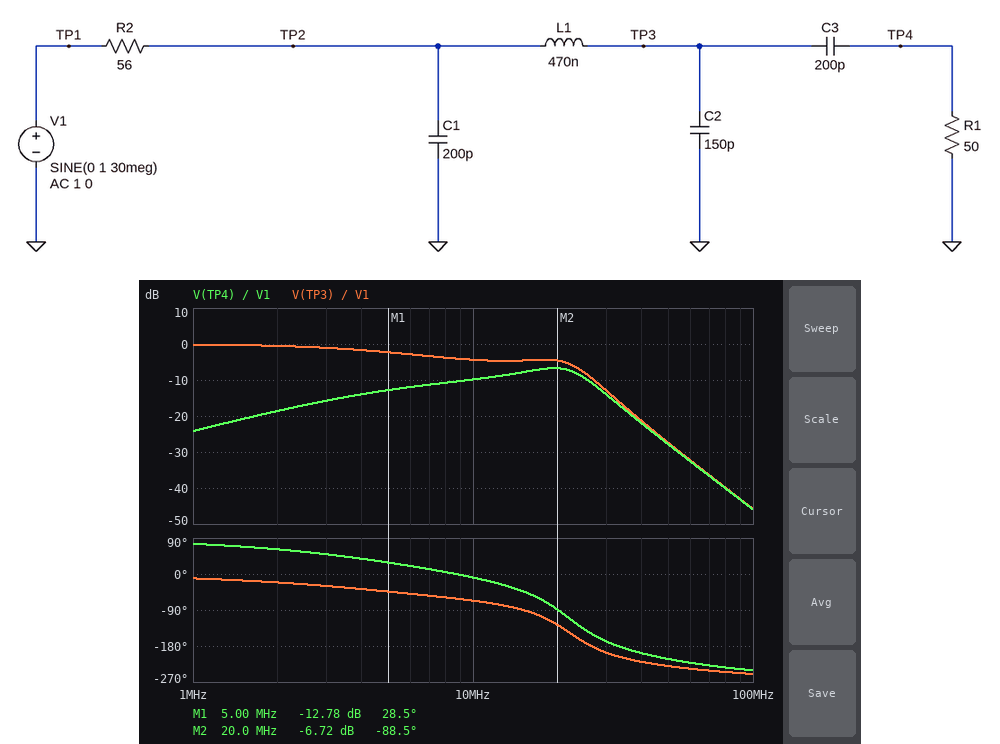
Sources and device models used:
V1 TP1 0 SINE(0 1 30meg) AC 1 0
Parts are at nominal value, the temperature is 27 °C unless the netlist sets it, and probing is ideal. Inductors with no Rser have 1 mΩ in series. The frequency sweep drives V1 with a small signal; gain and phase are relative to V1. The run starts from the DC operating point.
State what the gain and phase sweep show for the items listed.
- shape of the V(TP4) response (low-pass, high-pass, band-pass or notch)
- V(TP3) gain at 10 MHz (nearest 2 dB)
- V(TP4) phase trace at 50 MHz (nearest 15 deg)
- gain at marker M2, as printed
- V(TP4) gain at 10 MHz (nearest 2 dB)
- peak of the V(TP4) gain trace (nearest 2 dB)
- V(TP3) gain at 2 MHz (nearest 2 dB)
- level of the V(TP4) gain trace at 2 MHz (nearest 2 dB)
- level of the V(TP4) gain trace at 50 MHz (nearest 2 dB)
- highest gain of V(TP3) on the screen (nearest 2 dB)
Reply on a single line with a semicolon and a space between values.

band-pass; -4 dB; -210 deg; -6.72 dB; -10 dB; -6 dB; 0 dB; -18 dB; -28 dB; 0 dB
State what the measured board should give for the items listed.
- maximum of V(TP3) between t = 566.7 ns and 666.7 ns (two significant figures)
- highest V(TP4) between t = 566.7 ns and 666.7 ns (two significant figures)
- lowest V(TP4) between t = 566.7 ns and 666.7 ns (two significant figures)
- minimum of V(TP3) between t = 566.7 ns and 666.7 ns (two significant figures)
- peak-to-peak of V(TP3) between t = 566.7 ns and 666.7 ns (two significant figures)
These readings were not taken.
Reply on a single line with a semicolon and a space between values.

220 mV; 200 mV; -200 mV; -220 mV; 450 mV
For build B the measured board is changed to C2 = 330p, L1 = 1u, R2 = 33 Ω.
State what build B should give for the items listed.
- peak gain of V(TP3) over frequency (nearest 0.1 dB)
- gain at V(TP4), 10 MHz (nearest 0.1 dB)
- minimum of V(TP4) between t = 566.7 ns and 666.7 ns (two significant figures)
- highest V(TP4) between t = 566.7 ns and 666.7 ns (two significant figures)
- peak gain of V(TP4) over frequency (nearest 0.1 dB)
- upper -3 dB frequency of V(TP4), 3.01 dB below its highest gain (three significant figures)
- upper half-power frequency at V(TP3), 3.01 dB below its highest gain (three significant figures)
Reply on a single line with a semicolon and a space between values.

1.3 dB; -7.6 dB; -48 mV; 48 mV; -6.5 dB; 11.8 MHz; 9.72 MHz
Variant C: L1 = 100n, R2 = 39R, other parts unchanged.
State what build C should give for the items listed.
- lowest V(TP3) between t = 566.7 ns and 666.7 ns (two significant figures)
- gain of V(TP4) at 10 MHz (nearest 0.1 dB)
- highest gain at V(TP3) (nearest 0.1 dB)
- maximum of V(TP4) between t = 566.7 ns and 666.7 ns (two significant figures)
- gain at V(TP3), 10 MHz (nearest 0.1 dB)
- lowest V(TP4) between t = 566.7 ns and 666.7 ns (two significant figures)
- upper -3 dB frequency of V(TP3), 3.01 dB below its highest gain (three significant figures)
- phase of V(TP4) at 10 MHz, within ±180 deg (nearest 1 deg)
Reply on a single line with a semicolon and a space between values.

-450 mV; -9.6 dB; 0 dB; 400 mV; -4.1 dB; -400 mV; 7.45 MHz; 10 deg
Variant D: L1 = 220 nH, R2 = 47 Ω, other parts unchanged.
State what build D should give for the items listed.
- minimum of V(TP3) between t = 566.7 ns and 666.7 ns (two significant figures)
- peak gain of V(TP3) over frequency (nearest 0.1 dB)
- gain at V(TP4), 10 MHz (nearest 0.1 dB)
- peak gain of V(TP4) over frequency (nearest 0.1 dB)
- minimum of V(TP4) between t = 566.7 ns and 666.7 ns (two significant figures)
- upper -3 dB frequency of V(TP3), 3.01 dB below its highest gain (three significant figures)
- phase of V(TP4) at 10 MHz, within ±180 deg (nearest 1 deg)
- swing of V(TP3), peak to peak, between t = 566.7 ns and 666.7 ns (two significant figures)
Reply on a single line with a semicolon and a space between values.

-580 mV; 0 dB; -10.0 dB; -5.8 dB; -510 mV; 6.60 MHz; 3 deg; 1.2 V
